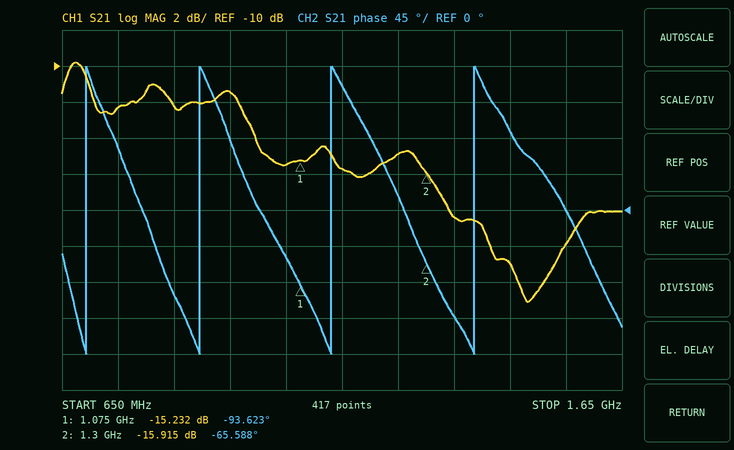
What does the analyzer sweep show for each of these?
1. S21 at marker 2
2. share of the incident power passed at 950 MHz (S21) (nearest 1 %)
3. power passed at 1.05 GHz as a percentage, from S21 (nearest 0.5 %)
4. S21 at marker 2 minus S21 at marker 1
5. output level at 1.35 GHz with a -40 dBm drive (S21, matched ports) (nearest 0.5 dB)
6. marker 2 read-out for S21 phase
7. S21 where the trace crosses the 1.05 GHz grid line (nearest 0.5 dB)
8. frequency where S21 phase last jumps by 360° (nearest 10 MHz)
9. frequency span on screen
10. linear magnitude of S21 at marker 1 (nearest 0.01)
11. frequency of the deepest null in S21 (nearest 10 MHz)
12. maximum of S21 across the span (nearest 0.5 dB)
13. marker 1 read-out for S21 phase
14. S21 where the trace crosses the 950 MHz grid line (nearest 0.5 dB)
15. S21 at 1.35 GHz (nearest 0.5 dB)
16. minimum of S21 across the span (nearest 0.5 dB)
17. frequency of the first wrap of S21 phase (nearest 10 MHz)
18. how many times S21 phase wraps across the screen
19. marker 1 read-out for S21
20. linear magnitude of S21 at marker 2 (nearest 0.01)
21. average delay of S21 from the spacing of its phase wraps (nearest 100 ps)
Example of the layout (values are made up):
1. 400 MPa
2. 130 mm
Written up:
1. -15.915 dB
2. 7 %
3. 3.0 %
4. -0.683 dB
5. -58.5 dBm
6. -65.588°
7. -15.5 dB
8. 1.39 GHz
9. 1 GHz
10. 0.17
11. 1.48 GHz
12. -10.0 dB
13. -93.623°
14. -11.5 dB
15. -18.5 dB
16. -23.0 dB
17. 690 MHz
18. 4
19. -15.232 dB
20. 0.16
21. 4.3 ns
